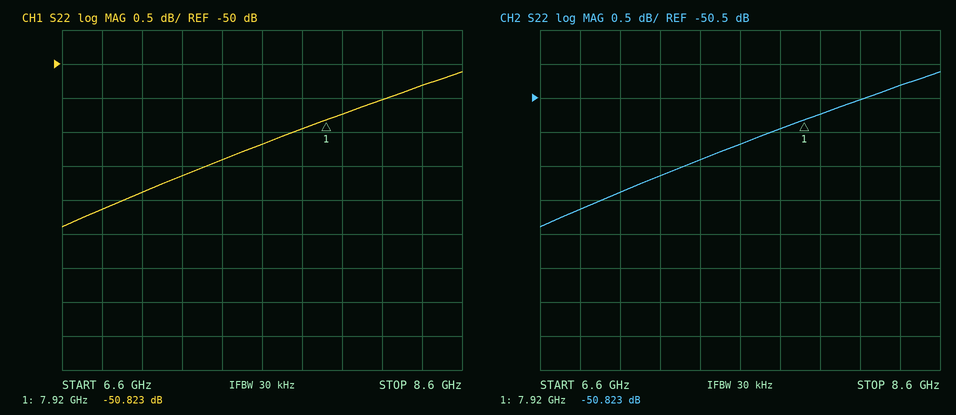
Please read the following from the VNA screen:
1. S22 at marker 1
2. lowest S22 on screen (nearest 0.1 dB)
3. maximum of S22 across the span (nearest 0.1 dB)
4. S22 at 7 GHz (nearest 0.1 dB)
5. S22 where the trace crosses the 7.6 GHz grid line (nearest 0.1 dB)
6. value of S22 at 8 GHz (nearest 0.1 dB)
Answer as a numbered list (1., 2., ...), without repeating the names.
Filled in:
1. -50.823 dB
2. -52.4 dB
3. -50.1 dB
4. -51.9 dB
5. -51.2 dB
6. -50.7 dB
